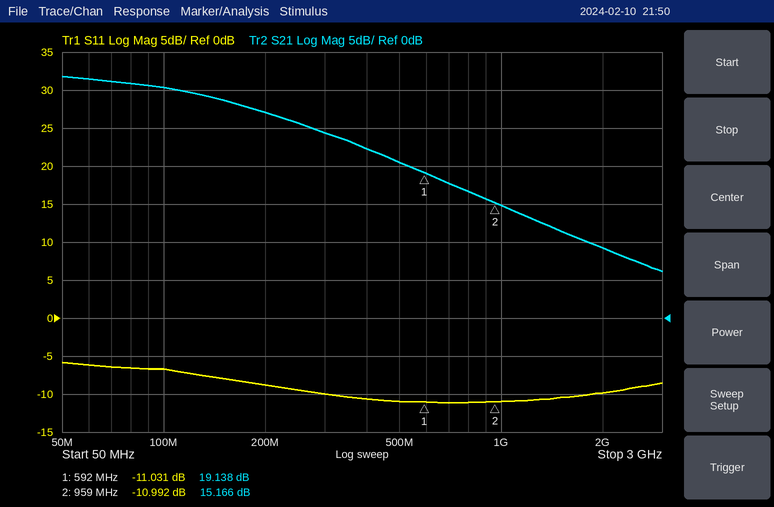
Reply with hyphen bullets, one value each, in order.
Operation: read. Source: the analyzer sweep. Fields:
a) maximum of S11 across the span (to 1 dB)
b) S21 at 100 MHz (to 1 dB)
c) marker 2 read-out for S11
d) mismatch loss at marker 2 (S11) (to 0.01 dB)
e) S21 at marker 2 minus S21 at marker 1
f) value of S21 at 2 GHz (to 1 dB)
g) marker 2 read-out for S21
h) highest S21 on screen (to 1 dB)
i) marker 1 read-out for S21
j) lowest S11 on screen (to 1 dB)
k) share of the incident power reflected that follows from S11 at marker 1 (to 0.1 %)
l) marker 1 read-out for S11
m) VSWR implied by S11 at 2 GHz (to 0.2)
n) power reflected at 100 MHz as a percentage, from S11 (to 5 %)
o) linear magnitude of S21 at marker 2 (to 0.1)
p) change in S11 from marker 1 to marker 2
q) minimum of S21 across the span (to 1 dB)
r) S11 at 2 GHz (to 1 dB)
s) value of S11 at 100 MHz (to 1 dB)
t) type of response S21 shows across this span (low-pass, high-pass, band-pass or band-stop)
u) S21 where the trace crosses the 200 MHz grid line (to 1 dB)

- -6 dB
- 30 dB
- -10.992 dB
- 0.36 dB
- -3.972 dB
- 9 dB
- 15.166 dB
- 32 dB
- 19.138 dB
- -11 dB
- 7.9 %
- -11.031 dB
- 2.0
- 20 %
- 5.7
- 0.039 dB
- 6 dB
- -10 dB
- -7 dB
- low-pass
- 27 dB
